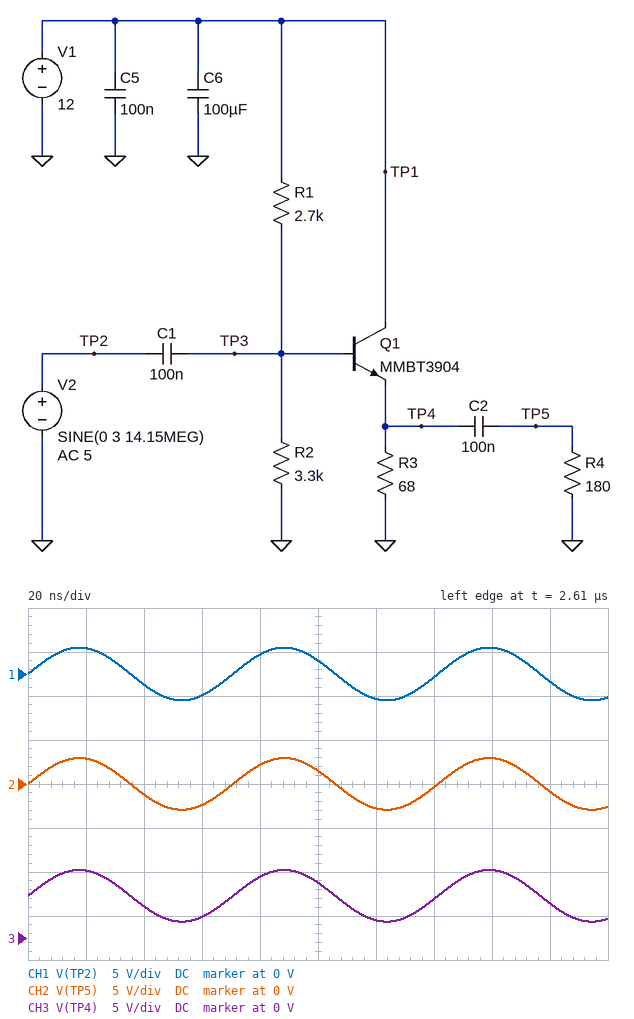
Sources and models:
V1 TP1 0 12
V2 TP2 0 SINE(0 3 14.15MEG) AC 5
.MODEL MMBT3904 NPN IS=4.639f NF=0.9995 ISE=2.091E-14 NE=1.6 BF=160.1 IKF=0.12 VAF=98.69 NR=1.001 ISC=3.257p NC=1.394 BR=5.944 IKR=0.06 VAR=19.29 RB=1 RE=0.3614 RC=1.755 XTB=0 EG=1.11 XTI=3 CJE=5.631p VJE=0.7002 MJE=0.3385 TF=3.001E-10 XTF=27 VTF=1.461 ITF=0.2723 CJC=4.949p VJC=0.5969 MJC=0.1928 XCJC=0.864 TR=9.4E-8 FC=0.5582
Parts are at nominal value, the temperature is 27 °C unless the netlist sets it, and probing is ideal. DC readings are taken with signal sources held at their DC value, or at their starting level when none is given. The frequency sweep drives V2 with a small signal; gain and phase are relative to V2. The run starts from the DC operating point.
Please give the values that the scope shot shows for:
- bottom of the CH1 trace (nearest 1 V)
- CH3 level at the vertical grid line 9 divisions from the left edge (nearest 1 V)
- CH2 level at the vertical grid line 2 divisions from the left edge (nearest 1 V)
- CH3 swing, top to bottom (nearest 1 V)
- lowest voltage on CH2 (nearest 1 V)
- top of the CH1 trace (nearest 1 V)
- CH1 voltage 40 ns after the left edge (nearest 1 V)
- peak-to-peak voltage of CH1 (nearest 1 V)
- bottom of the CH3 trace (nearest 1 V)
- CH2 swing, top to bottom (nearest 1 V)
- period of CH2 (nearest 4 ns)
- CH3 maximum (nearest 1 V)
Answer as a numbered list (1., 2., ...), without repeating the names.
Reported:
1. -3 V
2. 4 V
3. -1 V
4. 6 V
5. -3 V
6. 3 V
7. -1 V
8. 6 V
9. 2 V
10. 6 V
11. 72 ns
12. 8 V
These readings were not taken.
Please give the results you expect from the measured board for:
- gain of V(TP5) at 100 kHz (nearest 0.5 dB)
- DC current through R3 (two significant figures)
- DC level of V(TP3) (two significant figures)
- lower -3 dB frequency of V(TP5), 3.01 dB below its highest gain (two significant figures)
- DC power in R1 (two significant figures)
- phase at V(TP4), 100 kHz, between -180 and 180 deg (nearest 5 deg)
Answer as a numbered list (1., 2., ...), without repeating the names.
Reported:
1. 0 dB
2. 70 mA
3. 5.6 V
4. 9.1 kHz
5. 15 mW
6. 0 deg
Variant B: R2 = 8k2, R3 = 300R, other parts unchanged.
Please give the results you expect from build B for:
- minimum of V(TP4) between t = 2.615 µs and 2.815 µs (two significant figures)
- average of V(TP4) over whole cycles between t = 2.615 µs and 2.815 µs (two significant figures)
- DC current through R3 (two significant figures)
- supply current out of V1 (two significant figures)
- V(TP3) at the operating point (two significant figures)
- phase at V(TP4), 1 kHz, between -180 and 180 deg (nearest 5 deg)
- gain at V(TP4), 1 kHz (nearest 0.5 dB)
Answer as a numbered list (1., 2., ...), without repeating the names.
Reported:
1. 5.0 V
2. 7.9 V
3. 26 mA
4. 27 mA
5. 8.6 V
6. 40 deg
7. -2.5 dB
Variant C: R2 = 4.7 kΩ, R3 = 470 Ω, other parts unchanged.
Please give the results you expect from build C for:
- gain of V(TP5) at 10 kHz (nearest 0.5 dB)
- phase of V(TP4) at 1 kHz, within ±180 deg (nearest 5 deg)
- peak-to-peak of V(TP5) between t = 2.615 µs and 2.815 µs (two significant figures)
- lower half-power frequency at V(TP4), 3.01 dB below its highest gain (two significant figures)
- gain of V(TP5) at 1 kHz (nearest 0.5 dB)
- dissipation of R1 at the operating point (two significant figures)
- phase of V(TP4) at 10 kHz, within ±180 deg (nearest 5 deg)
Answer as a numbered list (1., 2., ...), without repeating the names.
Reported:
1. -2.5 dB
2. 45 deg
3. 5.0 V
4. 940 Hz
5. -22.0 dB
6. 7.7 mW
7. 5 deg
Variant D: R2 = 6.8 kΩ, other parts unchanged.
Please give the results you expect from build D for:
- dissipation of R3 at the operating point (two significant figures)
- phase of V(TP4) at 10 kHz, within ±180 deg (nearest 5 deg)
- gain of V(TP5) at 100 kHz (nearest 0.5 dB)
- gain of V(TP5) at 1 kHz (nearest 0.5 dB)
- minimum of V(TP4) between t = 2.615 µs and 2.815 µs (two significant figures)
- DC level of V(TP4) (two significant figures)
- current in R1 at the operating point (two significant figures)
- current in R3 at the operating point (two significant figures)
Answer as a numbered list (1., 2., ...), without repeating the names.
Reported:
1. 520 mW
2. 5 deg
3. 0 dB
4. -23.0 dB
5. 3.0 V
6. 6.0 V
7. 1.9 mA
8. 88 mA
